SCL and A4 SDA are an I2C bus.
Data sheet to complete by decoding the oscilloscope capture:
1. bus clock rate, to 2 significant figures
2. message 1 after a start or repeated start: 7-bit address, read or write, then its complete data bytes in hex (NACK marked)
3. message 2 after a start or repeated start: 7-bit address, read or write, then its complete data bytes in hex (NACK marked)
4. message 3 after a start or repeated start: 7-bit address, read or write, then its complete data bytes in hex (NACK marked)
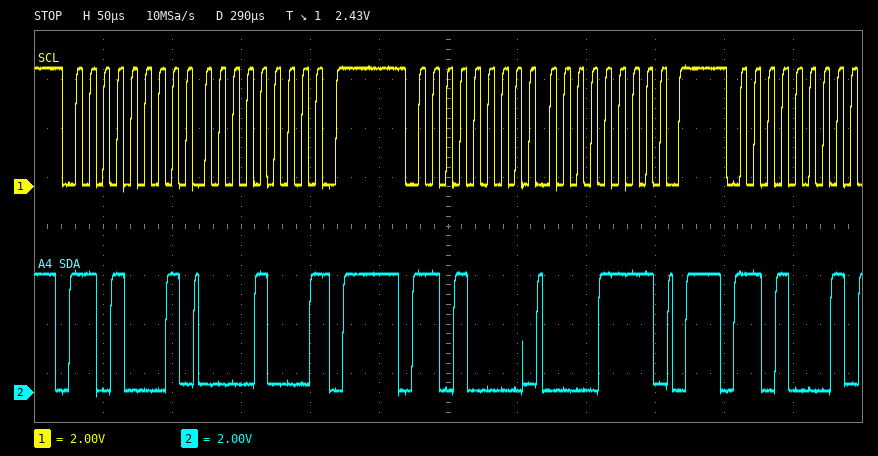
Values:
100 kHz
0x68 read: 08 NACK
0x68 write: 0F
0x68 read
